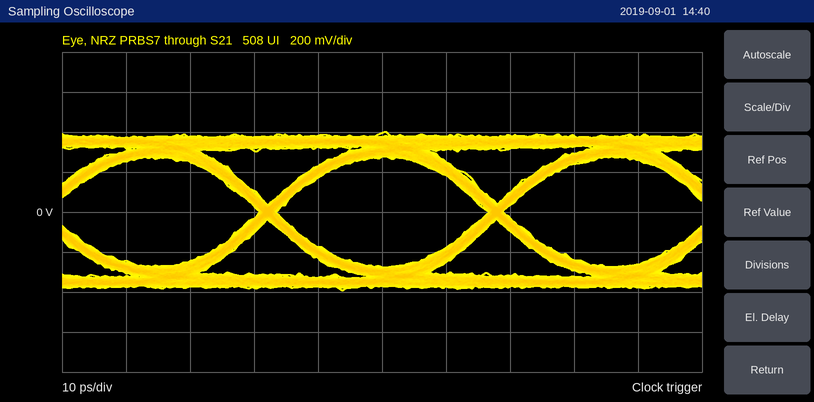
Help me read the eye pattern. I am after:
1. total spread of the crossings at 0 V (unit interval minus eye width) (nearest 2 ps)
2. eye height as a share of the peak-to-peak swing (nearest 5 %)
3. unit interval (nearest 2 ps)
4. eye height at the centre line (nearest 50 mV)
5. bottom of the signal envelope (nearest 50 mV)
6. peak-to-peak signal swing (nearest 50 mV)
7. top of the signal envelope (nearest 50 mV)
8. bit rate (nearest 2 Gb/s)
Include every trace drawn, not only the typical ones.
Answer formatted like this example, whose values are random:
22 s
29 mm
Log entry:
2 ps
70 %
36 ps
550 mV
-400 mV
800 mV
400 mV
28 Gb/s
